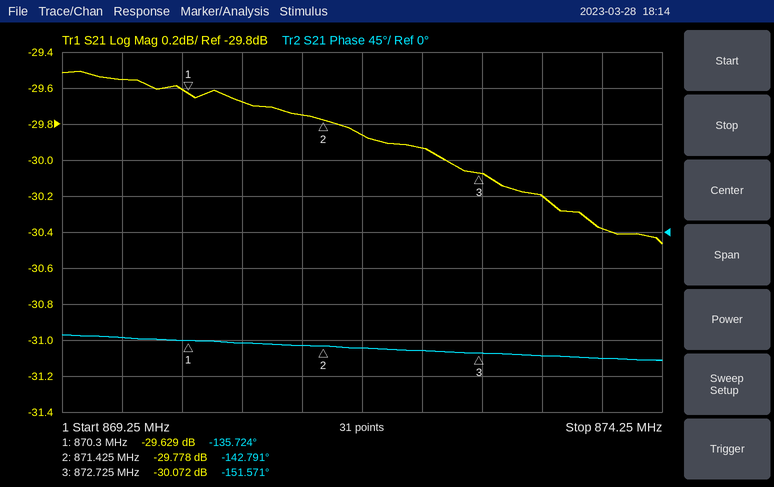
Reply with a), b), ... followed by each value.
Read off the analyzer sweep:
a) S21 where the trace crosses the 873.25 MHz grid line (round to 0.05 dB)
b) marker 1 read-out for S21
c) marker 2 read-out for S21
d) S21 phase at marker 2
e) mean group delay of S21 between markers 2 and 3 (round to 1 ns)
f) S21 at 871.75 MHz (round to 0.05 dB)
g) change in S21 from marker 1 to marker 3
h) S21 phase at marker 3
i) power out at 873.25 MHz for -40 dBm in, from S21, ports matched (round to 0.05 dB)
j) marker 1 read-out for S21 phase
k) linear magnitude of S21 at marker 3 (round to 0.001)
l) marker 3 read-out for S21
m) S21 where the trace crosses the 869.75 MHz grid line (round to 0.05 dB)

a) -30.20 dB
b) -29.629 dB
c) -29.778 dB
d) -142.791°
e) 19 ns
f) -29.85 dB
g) -0.443 dB
h) -151.571°
i) -70.20 dBm
j) -135.724°
k) 0.031
l) -30.072 dB
m) -29.55 dB
